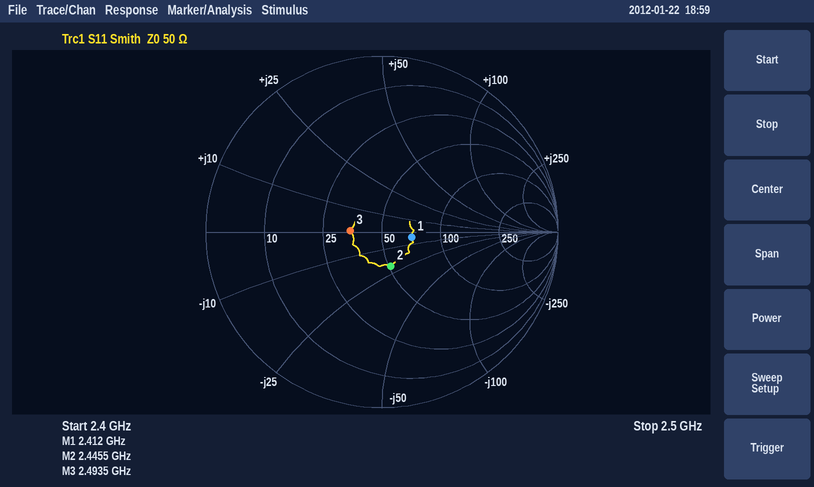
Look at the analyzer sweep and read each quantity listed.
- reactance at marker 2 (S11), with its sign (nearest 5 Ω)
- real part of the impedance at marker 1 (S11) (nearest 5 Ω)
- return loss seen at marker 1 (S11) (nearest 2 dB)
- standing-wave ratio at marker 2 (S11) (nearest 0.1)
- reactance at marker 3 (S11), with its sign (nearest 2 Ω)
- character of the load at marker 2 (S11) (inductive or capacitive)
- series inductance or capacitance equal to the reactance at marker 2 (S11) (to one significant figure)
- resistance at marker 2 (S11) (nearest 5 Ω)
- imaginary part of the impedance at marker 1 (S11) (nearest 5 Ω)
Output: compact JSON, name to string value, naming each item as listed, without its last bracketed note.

{"reactance at marker 2 (S11), with its sign": "-20 Ω", "real part of the impedance at marker 1 (S11)": "70 Ω", "return loss seen at marker 1 (S11)": "16 dB", "standing-wave ratio at marker 2 (S11)": "1.5", "reactance at marker 3 (S11), with its sign": "0 Ω", "character of the load at marker 2 (S11)": "capacitive", "series inductance or capacitance equal to the reactance at marker 2 (S11)": "3 pF", "resistance at marker 2 (S11)": "50 Ω", "imaginary part of the impedance at marker 1 (S11)": "-5 Ω"}
